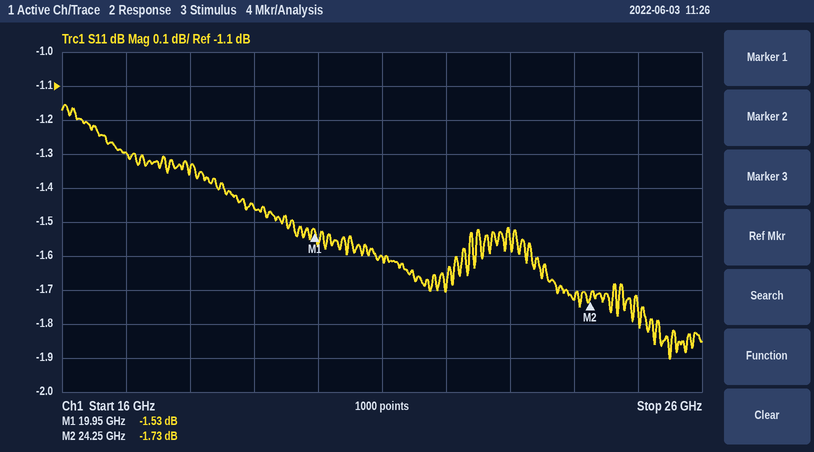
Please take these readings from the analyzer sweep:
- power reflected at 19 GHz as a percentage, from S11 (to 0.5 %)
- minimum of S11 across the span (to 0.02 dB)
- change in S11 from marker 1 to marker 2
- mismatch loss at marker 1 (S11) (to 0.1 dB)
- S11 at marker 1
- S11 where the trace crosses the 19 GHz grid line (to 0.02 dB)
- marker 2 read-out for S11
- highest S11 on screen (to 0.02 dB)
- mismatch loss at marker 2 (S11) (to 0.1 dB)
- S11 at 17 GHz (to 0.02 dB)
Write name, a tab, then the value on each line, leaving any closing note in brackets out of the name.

power reflected at 19 GHz as a percentage, from S11	71.5 %
minimum of S11 across the span	-1.90 dB
change in S11 from marker 1 to marker 2	-0.20 dB
mismatch loss at marker 1 (S11)	5.3 dB
S11 at marker 1	-1.53 dB
S11 where the trace crosses the 19 GHz grid line	-1.46 dB
marker 2 read-out for S11	-1.73 dB
highest S11 on screen	-1.16 dB
mismatch loss at marker 2 (S11)	4.8 dB
S11 at 17 GHz	-1.30 dB
